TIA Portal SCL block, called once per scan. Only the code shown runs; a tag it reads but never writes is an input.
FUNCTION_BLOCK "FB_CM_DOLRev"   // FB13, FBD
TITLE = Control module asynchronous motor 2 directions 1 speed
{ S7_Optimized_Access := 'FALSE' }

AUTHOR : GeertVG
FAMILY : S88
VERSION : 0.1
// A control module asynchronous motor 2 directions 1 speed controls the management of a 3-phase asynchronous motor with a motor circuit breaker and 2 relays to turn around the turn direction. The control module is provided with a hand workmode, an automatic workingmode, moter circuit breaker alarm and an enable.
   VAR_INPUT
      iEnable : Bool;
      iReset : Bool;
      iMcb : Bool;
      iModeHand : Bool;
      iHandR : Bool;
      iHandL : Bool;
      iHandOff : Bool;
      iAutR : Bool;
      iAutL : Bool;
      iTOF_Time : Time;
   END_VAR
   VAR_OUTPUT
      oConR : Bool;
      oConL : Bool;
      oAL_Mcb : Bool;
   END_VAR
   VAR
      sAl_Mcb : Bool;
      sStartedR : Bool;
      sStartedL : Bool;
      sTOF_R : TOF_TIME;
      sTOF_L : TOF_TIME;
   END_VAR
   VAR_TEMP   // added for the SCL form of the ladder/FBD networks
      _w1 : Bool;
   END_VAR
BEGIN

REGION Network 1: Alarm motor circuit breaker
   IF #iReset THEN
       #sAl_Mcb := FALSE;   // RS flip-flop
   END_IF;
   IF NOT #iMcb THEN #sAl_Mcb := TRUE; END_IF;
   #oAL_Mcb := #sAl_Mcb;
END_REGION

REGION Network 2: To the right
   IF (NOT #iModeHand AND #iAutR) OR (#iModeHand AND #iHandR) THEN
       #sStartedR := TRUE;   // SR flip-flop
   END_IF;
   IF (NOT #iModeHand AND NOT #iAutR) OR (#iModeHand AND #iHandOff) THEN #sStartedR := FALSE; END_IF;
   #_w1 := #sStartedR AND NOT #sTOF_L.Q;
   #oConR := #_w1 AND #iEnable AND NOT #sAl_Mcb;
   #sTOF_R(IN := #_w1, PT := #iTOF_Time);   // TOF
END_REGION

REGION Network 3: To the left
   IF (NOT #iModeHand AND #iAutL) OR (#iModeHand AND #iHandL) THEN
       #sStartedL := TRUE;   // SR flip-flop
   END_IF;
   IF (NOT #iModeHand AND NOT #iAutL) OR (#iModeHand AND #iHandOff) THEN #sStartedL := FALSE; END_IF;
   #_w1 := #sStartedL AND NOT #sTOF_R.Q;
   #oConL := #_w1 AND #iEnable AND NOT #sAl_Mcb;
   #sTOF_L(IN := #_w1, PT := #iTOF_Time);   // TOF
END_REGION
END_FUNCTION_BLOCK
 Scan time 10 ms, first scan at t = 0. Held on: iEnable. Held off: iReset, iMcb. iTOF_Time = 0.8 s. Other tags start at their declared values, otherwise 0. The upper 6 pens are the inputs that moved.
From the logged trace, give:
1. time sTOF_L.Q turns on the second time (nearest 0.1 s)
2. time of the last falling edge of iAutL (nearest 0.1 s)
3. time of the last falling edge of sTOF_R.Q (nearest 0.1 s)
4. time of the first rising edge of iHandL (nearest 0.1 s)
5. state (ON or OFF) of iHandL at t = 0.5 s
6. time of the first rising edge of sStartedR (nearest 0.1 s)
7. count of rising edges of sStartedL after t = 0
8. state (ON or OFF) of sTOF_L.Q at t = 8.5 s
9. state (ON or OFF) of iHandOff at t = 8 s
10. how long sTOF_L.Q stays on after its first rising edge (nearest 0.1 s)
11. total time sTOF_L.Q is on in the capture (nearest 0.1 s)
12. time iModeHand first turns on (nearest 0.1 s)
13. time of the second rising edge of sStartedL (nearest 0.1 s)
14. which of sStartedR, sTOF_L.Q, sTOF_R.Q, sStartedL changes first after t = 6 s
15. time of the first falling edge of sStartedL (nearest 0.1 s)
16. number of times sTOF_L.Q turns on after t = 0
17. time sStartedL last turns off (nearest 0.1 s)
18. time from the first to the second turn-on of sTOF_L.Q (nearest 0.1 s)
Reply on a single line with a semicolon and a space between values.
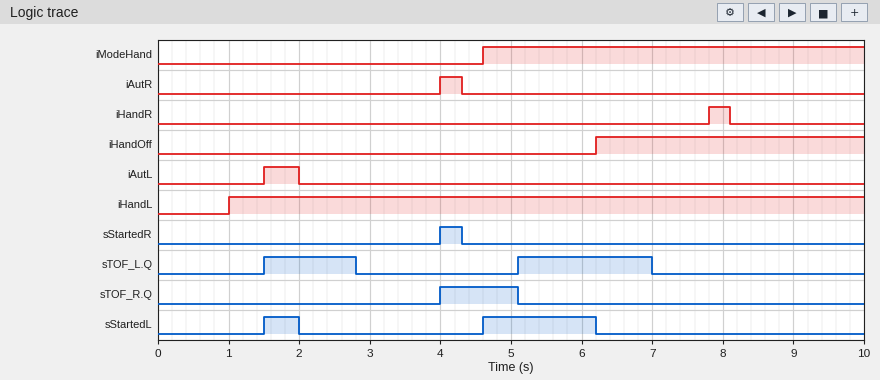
5.1 s; 2.0 s; 5.1 s; 1.0 s; OFF; 4.0 s; 2; OFF; ON; 1.3 s; 3.2 s; 4.6 s; 4.6 s; sStartedL; 2.0 s; 2; 6.2 s; 3.6 s
